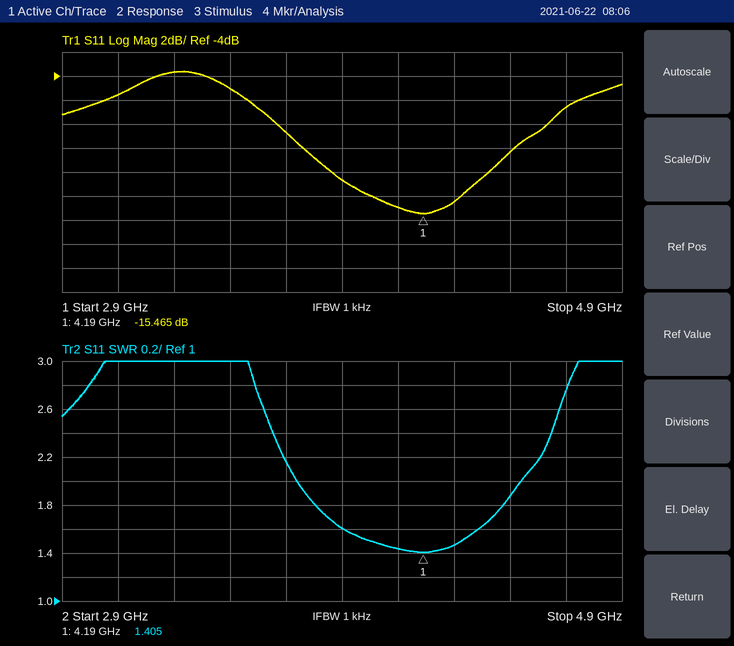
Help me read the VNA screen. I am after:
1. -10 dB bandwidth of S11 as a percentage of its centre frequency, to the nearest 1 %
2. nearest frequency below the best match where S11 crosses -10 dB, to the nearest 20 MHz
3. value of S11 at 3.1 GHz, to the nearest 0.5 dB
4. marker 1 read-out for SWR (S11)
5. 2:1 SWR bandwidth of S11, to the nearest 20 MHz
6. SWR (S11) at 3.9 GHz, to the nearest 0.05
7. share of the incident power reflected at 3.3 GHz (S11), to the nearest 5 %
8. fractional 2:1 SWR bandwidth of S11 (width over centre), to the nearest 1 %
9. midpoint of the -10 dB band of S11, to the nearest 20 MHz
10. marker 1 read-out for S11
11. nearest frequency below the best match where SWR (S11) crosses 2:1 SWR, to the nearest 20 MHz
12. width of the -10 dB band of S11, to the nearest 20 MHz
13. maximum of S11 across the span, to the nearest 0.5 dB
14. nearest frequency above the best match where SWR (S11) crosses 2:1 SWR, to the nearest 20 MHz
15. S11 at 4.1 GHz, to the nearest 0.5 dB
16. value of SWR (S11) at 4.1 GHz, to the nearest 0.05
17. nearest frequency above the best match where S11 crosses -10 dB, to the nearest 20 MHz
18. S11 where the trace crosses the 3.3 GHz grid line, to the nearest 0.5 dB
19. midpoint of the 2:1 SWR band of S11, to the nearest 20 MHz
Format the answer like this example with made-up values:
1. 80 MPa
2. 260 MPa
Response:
1. 18 %
2. 3.76 GHz
3. -5.5 dB
4. 1.405
5. 800 MHz
6. 1.60
7. 45 %
8. 19 %
9. 4.14 GHz
10. -15.465 dB
11. 3.74 GHz
12. 760 MHz
13. -3.5 dB
14. 4.54 GHz
15. -15.0 dB
16. 1.45
17. 4.52 GHz
18. -3.5 dB
19. 4.14 GHz
